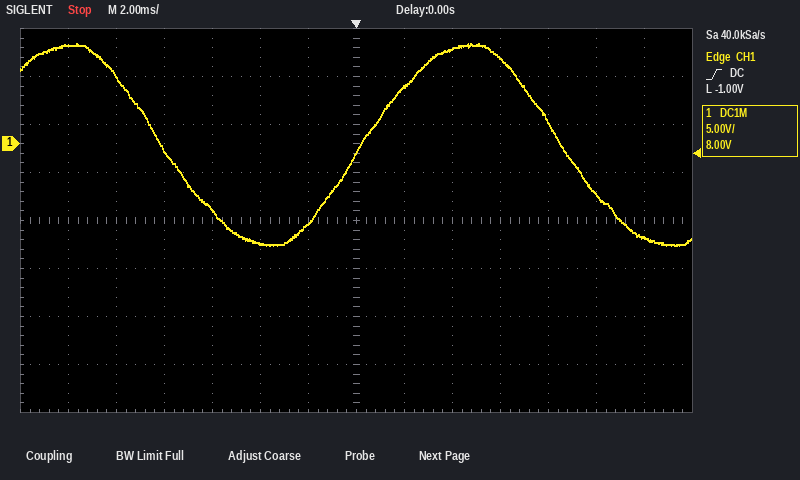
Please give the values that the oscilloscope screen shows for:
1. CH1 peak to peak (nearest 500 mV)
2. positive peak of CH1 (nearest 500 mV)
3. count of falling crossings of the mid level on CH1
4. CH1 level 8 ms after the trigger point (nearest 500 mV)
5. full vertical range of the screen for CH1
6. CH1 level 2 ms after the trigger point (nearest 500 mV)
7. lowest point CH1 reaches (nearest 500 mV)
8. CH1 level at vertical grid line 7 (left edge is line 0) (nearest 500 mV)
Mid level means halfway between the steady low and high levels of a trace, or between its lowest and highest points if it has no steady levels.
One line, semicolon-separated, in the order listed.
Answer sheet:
21.0 V; 10.5 V; 2; 2.5 V; 40 V; 6.0 V; -10.5 V; -1.0 V
